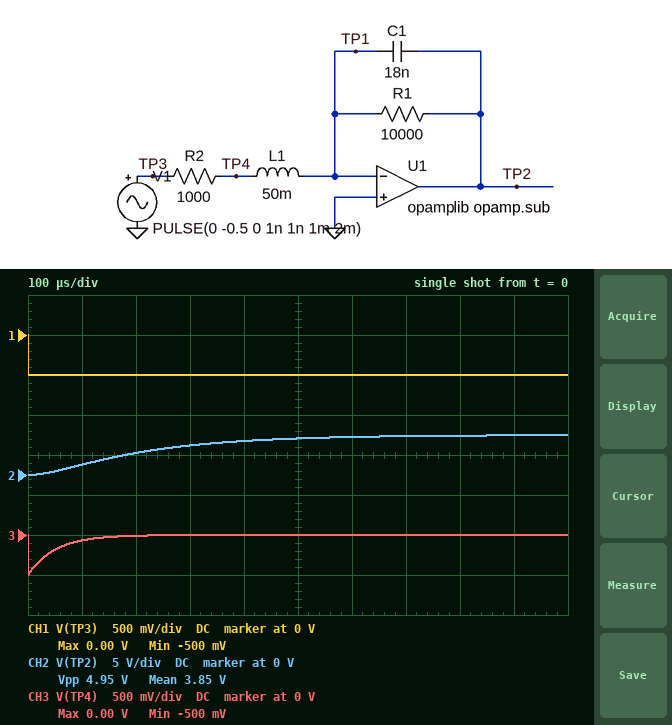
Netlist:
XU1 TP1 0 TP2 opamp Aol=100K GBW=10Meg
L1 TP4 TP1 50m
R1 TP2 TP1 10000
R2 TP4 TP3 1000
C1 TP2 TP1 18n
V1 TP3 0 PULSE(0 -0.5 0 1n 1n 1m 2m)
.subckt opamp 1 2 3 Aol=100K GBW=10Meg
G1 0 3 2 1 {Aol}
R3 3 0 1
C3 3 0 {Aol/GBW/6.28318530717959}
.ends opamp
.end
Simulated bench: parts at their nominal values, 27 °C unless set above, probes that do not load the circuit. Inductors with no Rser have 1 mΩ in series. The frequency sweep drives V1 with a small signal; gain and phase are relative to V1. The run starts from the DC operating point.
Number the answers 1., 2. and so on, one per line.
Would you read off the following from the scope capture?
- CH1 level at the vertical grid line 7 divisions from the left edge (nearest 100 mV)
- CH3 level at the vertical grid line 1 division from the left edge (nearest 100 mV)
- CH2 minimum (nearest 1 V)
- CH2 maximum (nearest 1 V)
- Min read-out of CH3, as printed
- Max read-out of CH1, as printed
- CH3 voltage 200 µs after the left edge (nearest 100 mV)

1. -500 mV
2. -100 mV
3. 0 V
4. 5 V
5. -500 mV
6. 0.00 V
7. 0 V
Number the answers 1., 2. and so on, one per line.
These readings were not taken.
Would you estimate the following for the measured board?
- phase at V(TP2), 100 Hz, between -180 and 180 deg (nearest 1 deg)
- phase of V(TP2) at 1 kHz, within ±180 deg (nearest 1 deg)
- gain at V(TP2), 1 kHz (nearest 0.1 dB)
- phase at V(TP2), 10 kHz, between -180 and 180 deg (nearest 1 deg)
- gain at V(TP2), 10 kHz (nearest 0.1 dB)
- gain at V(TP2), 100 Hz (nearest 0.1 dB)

1. 172 deg
2. 114 deg
3. 16.0 dB
4. 23 deg
5. -11.5 dB
6. 19.9 dB
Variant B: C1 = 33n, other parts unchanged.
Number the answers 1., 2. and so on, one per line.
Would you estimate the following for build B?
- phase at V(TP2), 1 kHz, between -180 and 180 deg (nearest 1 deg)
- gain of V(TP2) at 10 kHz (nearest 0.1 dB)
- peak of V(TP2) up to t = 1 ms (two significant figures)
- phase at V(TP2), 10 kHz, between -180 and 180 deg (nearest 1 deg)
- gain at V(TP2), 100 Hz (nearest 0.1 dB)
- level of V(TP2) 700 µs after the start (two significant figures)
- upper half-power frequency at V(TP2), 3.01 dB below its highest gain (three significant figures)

1. 98 deg
2. -16.7 dB
3. 4.7 V
4. 20 deg
5. 19.8 dB
6. 4.3 V
7. 472 Hz
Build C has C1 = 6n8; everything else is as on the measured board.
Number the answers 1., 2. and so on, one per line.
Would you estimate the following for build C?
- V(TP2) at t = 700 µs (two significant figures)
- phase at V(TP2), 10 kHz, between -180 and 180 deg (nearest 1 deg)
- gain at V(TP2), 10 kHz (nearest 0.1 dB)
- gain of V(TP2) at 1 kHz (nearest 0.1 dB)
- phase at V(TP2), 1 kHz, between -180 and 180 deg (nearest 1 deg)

1. 5.0 V
2. 31 deg
3. -3.2 dB
4. 18.9 dB
5. 139 deg
